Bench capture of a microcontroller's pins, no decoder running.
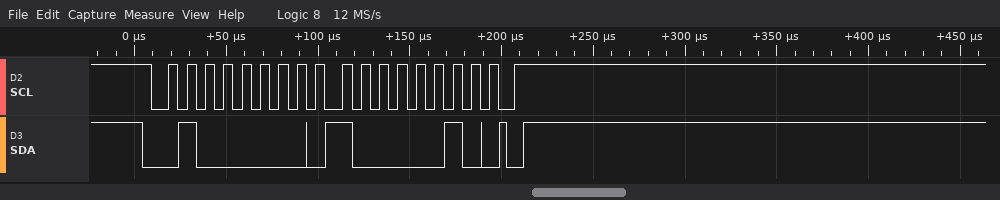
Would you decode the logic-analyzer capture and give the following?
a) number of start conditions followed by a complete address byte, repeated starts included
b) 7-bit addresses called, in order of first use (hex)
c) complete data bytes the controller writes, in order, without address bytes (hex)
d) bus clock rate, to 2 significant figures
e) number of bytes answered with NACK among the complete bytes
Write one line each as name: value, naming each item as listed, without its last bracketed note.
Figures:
number of start conditions followed by a complete address byte, repeated starts included: 1
7-bit addresses called, in order of first use: 0x20
complete data bytes the controller writes, in order, without address bytes: 82
bus clock rate, to 2 significant figures: 100 kHz
number of bytes answered with NACK among the complete bytes: 0
